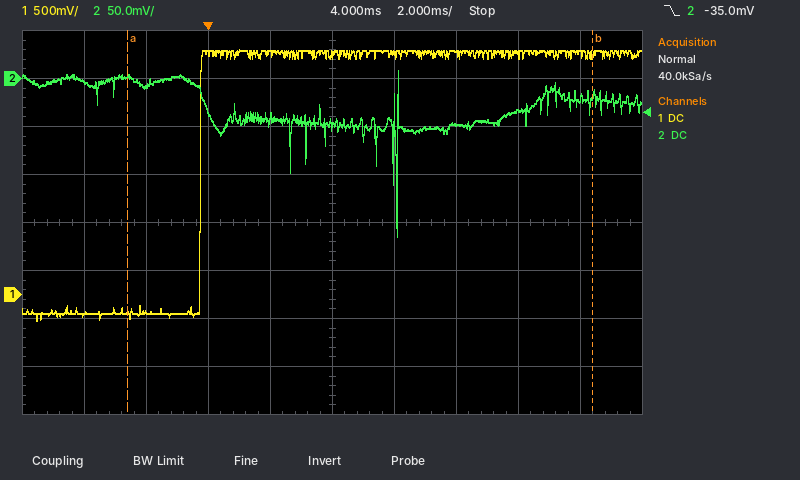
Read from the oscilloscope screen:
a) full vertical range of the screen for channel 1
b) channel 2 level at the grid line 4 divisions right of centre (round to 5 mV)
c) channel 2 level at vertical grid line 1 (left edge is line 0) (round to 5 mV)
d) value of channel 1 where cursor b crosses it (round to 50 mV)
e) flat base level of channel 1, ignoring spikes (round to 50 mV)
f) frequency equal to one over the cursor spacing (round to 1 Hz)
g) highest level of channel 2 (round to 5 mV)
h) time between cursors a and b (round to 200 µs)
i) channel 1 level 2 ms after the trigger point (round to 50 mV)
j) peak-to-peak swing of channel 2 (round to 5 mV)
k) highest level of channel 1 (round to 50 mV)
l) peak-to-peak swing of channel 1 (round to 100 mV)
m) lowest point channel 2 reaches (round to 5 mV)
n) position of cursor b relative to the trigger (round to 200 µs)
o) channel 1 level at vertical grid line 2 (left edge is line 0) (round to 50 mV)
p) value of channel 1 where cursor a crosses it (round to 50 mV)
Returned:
4 V
-20 mV
-5 mV
2.50 V
-200 mV
67 Hz
10 mV
15.0 ms
2.50 V
175 mV
2.55 V
2.80 V
-165 mV
+12.4 ms
-200 mV
-200 mV
